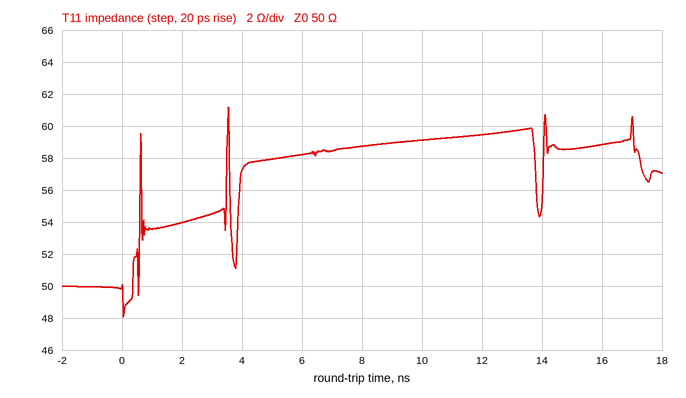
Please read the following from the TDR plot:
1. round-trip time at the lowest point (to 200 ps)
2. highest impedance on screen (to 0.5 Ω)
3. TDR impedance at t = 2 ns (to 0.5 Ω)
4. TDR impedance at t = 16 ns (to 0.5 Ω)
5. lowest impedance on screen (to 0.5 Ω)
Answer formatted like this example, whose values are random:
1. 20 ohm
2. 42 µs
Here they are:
1. 0.0 ns
2. 61.0 Ω
3. 54.0 Ω
4. 59.0 Ω
5. 48.0 Ω
